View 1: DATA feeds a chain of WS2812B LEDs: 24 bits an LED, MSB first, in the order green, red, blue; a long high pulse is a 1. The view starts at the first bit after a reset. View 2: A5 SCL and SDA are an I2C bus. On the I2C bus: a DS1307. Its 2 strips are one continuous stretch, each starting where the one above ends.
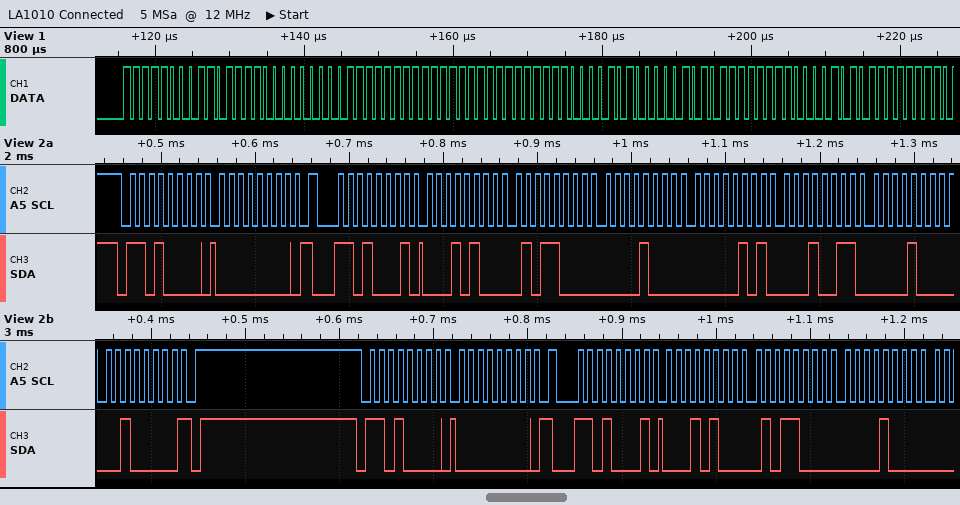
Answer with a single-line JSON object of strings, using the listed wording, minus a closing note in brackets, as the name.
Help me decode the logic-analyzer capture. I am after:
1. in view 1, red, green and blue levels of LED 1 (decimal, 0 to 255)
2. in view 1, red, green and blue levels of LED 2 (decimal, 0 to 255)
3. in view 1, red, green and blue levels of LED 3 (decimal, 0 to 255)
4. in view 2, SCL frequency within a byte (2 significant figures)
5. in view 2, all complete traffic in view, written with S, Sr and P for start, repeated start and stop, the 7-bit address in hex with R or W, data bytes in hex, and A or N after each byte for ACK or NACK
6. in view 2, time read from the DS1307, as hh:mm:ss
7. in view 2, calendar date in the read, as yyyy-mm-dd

{"in view 1, red, green and blue levels of LED 1": "222, 248, 0", "in view 1, red, green and blue levels of LED 2": "255, 255, 255", "in view 1, red, green and blue levels of LED 3": "10, 10, 255", "in view 2, SCL frequency within a byte": "100 kHz", "in view 2, all complete traffic in view, written with S, Sr and P for start, repeated start and stop, the 7-bit address in hex with R or W, data bytes in hex, and A or N after each byte for ACK or NACK": "S 68W A 00 A Sr 68R A 14 A 58 A 08 A 05 A 13 A 08 A 20 N P S 68W A 00 A Sr 68R A 14 A 58 A 08 A", "in view 2, time read from the DS1307, as hh:mm:ss": "08:58:14", "in view 2, calendar date in the read, as yyyy-mm-dd": "2020-08-13"}
